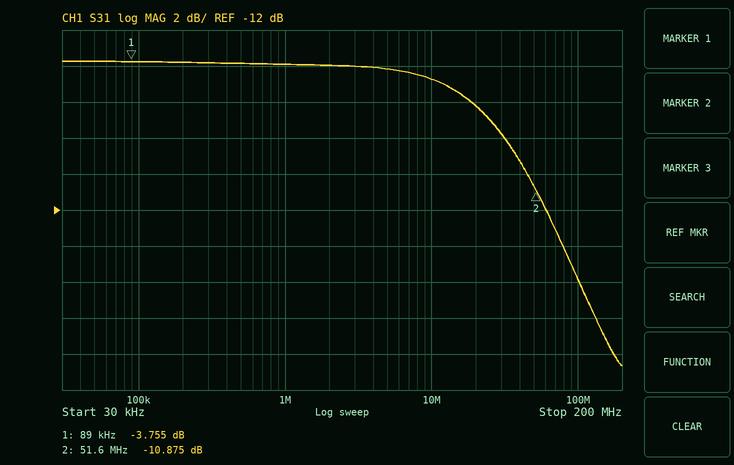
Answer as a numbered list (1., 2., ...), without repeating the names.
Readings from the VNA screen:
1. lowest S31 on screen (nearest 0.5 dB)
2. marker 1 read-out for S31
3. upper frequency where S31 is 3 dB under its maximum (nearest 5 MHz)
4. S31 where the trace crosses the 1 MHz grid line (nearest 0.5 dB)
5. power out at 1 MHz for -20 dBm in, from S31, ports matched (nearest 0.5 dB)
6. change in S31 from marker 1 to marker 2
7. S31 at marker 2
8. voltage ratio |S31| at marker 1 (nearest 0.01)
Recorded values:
1. -20.5 dB
2. -3.755 dB
3. 25 MHz
4. -4.0 dB
5. -24.0 dBm
6. -7.120 dB
7. -10.875 dB
8. 0.65
